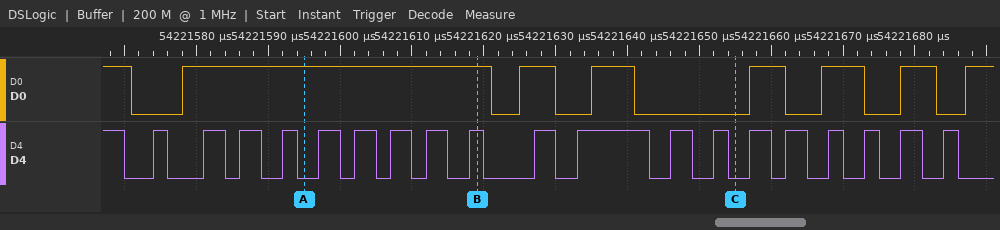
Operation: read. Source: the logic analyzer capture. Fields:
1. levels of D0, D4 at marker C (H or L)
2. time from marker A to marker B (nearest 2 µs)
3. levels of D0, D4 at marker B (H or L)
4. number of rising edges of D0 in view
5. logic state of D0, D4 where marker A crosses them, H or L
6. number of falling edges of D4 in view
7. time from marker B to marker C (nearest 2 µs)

D0=L, D4=L
24 µs
D0=H, D4=H
7
D0=H, D4=L
20
36 µs
